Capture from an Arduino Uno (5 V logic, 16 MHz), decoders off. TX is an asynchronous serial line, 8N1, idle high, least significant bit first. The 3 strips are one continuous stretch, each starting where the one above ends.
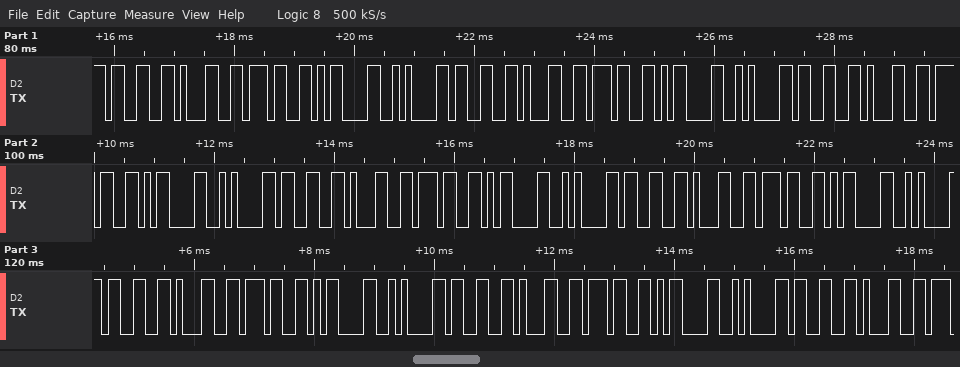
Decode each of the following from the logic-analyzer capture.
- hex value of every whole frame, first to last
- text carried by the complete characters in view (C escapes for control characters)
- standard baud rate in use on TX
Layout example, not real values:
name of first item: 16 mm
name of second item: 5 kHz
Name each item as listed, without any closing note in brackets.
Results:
hex value of every whole frame, first to last: 33 31 37 0D 0A 33 31 37 0D 0A 33 31 37 0D 0A 33 31 37 0D 0A 33 31 37 0D 0A 33 31 37 0D 0A 33 31 37 0D 0A 33 31
text carried by the complete characters in view: "317\r\n317\r\n317\r\n317\r\n317\r\n317\r\n317\r\n31"
standard baud rate in use on TX: 9600 baud
